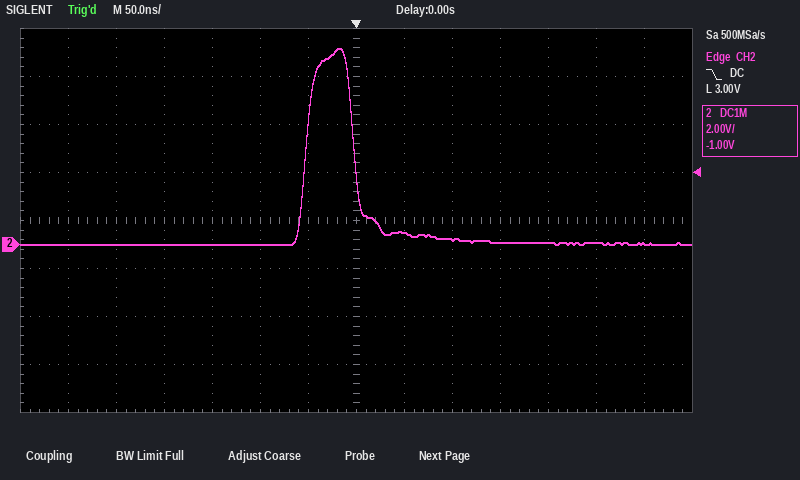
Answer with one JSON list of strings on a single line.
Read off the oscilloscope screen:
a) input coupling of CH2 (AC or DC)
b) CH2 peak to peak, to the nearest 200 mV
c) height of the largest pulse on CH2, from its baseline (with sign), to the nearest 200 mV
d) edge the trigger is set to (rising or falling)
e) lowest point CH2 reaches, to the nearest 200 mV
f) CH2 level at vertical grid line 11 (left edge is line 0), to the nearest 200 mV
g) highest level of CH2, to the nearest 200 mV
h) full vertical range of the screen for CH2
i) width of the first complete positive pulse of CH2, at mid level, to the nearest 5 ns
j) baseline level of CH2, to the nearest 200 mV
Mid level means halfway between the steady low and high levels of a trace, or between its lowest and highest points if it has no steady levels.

["DC", "8.2 V", "+8.2 V", "falling", "0.0 V", "0.0 V", "8.2 V", "16 V", "50 ns", "0.0 V"]
